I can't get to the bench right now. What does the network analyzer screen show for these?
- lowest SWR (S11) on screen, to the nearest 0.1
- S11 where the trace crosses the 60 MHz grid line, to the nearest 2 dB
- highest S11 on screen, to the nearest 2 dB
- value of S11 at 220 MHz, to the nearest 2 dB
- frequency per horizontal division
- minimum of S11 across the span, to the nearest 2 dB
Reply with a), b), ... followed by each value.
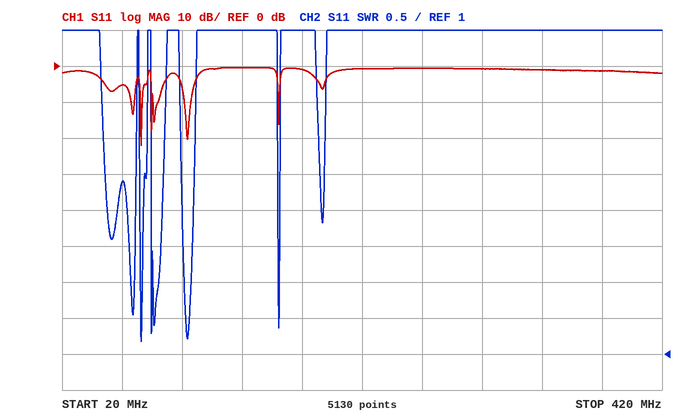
a) 1.2
b) -6 dB
c) 0 dB
d) 0 dB
e) 40 MHz
f) -22 dB
